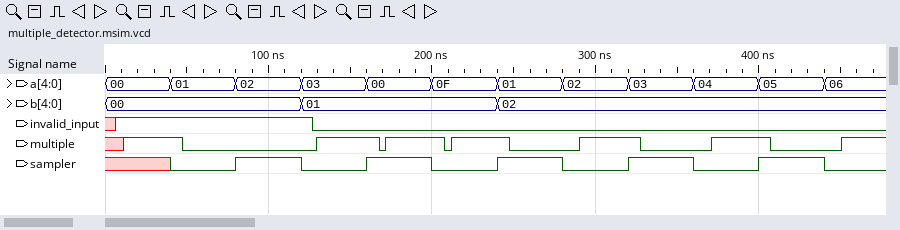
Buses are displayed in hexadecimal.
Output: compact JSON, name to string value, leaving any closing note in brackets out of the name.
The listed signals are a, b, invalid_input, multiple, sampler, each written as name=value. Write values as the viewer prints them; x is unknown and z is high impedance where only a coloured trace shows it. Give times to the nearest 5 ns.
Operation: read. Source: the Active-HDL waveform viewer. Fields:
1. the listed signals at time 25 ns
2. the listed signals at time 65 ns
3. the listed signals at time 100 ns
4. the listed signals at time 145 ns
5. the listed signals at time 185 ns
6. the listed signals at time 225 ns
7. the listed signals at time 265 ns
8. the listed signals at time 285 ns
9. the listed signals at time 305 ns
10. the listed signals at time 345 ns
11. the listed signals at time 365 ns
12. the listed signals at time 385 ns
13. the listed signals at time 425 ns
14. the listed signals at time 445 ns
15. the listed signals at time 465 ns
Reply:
{"the listed signals at time 25 ns": "a=00, b=00, invalid_input=1, multiple=1, sampler=x", "the listed signals at time 65 ns": "a=01, b=00, invalid_input=1, multiple=0, sampler=0", "the listed signals at time 100 ns": "a=02, b=00, invalid_input=1, multiple=0, sampler=1", "the listed signals at time 145 ns": "a=03, b=01, invalid_input=0, multiple=1, sampler=0", "the listed signals at time 185 ns": "a=00, b=01, invalid_input=0, multiple=1, sampler=1", "the listed signals at time 225 ns": "a=0F, b=01, invalid_input=0, multiple=1, sampler=0", "the listed signals at time 265 ns": "a=01, b=02, invalid_input=0, multiple=0, sampler=1", "the listed signals at time 285 ns": "a=02, b=02, invalid_input=0, multiple=0, sampler=0", "the listed signals at time 305 ns": "a=02, b=02, invalid_input=0, multiple=1, sampler=0", "the listed signals at time 345 ns": "a=03, b=02, invalid_input=0, multiple=0, sampler=1", "the listed signals at time 365 ns": "a=04, b=02, invalid_input=0, multiple=0, sampler=0", "the listed signals at time 385 ns": "a=04, b=02, invalid_input=0, multiple=1, sampler=0", "the listed signals at time 425 ns": "a=05, b=02, invalid_input=0, multiple=0, sampler=1", "the listed signals at time 445 ns": "a=06, b=02, invalid_input=0, multiple=0, sampler=0", "the listed signals at time 465 ns": "a=06, b=02, invalid_input=0, multiple=1, sampler=0"}
